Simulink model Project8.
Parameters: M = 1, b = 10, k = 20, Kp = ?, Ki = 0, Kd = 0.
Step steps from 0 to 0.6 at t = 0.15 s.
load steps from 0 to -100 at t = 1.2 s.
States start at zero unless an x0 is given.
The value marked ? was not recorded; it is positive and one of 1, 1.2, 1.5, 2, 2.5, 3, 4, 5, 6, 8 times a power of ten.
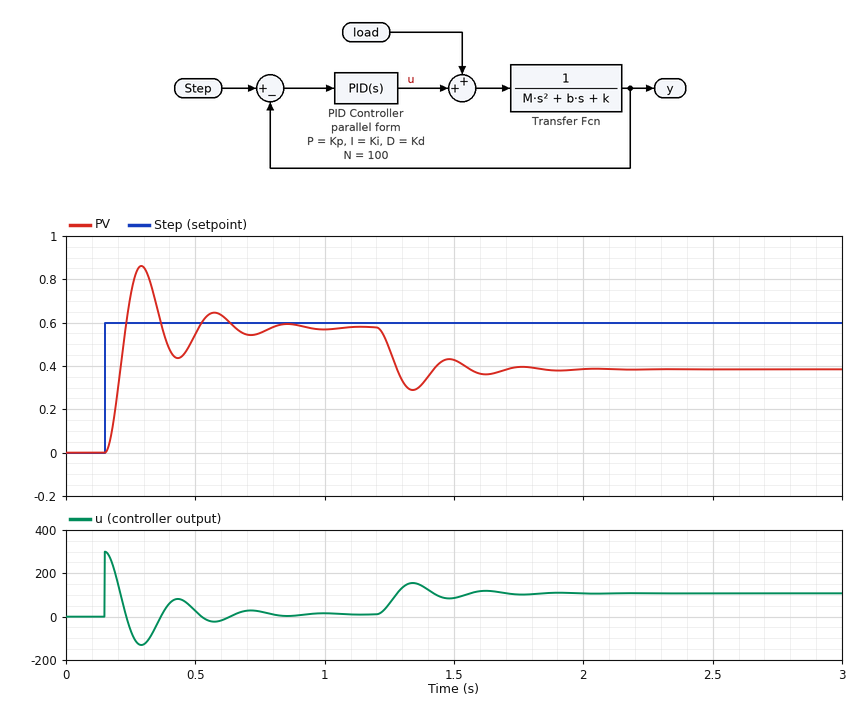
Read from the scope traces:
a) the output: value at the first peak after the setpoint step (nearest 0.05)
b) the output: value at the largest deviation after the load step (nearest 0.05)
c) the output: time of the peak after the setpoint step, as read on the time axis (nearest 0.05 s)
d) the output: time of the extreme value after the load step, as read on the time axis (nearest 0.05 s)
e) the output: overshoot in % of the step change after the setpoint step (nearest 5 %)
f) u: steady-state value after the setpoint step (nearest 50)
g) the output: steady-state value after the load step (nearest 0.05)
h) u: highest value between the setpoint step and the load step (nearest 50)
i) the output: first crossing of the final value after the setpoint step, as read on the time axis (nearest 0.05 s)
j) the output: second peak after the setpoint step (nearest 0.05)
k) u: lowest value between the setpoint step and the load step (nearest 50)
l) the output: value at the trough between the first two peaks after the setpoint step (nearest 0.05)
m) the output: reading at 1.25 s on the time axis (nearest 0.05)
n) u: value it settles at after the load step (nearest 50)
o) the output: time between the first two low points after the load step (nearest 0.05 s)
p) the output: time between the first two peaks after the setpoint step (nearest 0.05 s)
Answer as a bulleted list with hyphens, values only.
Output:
- 0.85
- 0.30
- 0.30 s
- 1.35 s
- 50 %
- 0
- 0.40
- 300
- 0.25 s
- 0.65
- -150
- 0.45
- 0.50
- 100
- 0.30 s
- 0.30 s
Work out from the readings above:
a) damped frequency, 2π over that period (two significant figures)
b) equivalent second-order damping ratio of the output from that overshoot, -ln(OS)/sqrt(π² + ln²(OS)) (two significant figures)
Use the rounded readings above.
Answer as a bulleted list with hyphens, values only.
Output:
- 21 rad/s
- 0.22
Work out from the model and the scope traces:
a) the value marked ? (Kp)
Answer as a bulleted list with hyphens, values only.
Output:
- 500
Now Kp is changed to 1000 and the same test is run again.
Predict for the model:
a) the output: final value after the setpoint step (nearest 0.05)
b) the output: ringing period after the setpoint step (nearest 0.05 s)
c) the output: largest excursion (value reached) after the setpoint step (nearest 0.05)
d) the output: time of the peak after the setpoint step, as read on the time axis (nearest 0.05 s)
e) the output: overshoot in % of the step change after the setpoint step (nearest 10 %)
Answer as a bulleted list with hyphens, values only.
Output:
- 0.60
- 0.20 s
- 0.95
- 0.25 s
- 60 %
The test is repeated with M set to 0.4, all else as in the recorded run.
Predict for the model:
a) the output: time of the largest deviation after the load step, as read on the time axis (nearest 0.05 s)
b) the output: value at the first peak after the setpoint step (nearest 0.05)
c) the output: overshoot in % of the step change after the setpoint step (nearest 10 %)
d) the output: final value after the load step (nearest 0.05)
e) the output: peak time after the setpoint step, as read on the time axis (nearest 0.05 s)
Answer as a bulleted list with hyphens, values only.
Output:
- 1.30 s
- 0.75
- 30 %
- 0.40
- 0.25 s
